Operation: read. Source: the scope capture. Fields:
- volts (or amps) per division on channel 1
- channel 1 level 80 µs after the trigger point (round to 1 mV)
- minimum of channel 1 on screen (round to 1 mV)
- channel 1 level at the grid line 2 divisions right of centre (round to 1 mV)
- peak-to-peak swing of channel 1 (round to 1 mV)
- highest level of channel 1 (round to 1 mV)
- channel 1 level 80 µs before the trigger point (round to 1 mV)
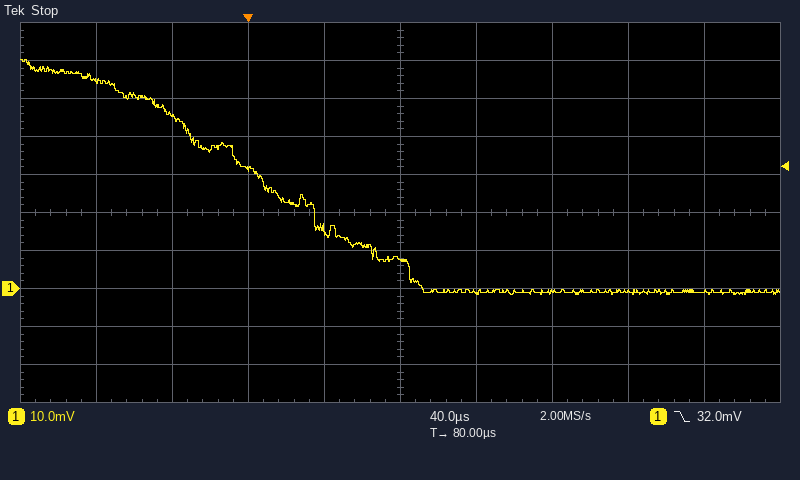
10 mV
8 mV
-2 mV
-1 mV
62 mV
60 mV
55 mV
